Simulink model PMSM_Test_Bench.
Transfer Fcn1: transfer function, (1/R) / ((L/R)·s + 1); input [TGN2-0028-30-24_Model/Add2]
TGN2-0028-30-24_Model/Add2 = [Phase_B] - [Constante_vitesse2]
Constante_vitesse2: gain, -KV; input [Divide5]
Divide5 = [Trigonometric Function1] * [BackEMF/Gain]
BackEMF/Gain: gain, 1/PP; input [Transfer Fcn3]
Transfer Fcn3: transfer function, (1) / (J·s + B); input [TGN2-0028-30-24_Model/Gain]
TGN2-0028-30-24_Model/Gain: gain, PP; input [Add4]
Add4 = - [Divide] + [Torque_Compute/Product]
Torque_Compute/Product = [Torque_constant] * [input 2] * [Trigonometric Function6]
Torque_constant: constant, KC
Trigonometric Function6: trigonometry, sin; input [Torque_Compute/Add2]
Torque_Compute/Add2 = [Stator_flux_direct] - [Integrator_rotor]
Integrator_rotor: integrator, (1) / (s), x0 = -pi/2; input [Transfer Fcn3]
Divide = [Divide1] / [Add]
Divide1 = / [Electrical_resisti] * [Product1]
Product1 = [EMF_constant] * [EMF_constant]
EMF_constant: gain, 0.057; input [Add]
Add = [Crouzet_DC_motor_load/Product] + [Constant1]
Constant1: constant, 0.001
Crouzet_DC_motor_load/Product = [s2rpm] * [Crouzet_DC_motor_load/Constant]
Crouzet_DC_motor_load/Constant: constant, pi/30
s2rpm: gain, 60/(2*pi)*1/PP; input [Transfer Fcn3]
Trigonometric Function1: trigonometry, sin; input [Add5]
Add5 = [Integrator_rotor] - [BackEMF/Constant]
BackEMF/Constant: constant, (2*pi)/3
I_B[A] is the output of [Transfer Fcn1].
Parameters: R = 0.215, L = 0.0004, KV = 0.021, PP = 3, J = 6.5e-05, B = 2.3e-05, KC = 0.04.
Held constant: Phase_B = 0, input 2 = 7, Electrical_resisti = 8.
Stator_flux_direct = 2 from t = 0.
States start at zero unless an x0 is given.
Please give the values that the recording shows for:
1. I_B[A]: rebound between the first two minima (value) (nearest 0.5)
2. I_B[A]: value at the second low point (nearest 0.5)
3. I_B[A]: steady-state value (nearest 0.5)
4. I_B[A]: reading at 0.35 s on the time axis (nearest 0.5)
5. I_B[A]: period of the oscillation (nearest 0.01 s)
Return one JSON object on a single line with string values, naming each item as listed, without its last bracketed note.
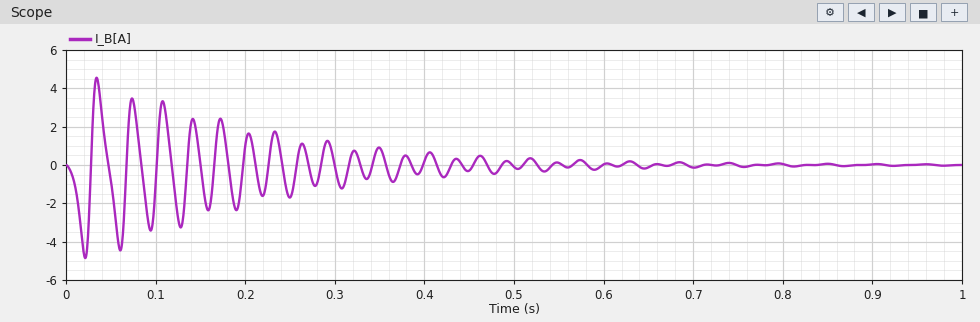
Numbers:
{"I_B[A]: rebound between the first two minima (value)": "4.5", "I_B[A]: value at the second low point": "-4.5", "I_B[A]: steady-state value": "0.0", "I_B[A]: reading at 0.35 s on the time axis": "1.0", "I_B[A]: period of the oscillation": "0.04 s"}
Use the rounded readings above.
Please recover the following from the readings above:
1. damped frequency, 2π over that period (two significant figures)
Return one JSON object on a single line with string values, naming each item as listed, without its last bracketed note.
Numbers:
{"damped frequency, 2π over that period": "160 rad/s"}
